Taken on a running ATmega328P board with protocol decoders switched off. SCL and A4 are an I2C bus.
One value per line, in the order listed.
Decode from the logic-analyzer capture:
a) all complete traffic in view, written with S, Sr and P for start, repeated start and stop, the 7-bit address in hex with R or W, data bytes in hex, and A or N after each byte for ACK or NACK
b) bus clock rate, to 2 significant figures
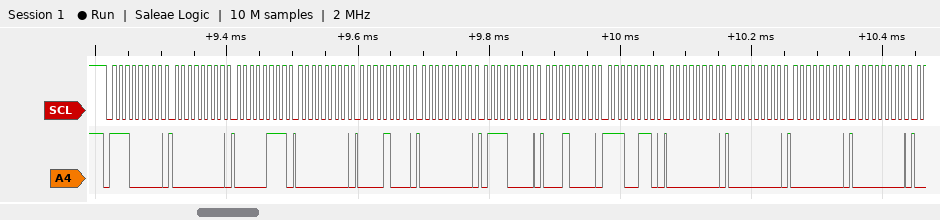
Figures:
S 70W A 00 A 07 A 00 A 08 A 00 A 70 A 10 A E6 A 00 A 00 A 00 A 00 A
100 kHz
